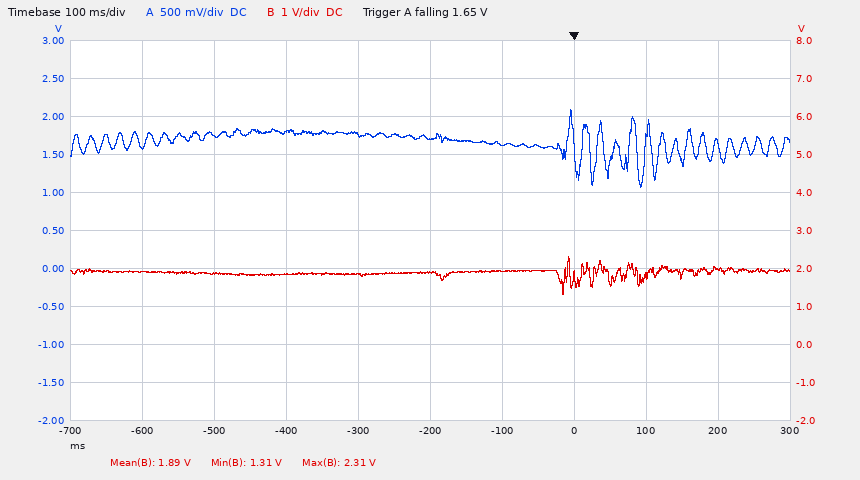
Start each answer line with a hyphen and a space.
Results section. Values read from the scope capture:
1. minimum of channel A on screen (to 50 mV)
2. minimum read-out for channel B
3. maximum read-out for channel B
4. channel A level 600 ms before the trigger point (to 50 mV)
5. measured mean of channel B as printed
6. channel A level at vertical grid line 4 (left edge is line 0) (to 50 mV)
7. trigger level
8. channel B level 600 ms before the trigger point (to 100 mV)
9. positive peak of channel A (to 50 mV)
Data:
- 1.05 V
- 1.31 V
- 2.31 V
- 1.60 V
- 1.89 V
- 1.75 V
- 1.65 V
- 1.9 V
- 2.10 V
